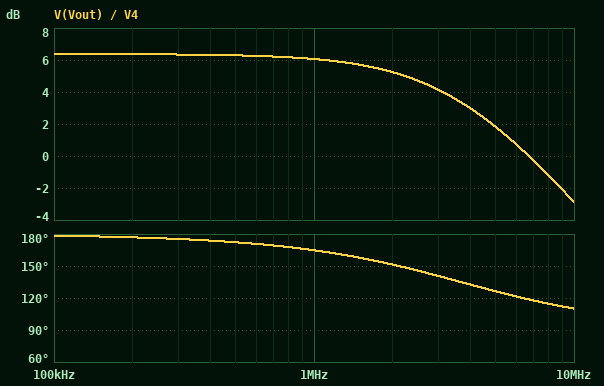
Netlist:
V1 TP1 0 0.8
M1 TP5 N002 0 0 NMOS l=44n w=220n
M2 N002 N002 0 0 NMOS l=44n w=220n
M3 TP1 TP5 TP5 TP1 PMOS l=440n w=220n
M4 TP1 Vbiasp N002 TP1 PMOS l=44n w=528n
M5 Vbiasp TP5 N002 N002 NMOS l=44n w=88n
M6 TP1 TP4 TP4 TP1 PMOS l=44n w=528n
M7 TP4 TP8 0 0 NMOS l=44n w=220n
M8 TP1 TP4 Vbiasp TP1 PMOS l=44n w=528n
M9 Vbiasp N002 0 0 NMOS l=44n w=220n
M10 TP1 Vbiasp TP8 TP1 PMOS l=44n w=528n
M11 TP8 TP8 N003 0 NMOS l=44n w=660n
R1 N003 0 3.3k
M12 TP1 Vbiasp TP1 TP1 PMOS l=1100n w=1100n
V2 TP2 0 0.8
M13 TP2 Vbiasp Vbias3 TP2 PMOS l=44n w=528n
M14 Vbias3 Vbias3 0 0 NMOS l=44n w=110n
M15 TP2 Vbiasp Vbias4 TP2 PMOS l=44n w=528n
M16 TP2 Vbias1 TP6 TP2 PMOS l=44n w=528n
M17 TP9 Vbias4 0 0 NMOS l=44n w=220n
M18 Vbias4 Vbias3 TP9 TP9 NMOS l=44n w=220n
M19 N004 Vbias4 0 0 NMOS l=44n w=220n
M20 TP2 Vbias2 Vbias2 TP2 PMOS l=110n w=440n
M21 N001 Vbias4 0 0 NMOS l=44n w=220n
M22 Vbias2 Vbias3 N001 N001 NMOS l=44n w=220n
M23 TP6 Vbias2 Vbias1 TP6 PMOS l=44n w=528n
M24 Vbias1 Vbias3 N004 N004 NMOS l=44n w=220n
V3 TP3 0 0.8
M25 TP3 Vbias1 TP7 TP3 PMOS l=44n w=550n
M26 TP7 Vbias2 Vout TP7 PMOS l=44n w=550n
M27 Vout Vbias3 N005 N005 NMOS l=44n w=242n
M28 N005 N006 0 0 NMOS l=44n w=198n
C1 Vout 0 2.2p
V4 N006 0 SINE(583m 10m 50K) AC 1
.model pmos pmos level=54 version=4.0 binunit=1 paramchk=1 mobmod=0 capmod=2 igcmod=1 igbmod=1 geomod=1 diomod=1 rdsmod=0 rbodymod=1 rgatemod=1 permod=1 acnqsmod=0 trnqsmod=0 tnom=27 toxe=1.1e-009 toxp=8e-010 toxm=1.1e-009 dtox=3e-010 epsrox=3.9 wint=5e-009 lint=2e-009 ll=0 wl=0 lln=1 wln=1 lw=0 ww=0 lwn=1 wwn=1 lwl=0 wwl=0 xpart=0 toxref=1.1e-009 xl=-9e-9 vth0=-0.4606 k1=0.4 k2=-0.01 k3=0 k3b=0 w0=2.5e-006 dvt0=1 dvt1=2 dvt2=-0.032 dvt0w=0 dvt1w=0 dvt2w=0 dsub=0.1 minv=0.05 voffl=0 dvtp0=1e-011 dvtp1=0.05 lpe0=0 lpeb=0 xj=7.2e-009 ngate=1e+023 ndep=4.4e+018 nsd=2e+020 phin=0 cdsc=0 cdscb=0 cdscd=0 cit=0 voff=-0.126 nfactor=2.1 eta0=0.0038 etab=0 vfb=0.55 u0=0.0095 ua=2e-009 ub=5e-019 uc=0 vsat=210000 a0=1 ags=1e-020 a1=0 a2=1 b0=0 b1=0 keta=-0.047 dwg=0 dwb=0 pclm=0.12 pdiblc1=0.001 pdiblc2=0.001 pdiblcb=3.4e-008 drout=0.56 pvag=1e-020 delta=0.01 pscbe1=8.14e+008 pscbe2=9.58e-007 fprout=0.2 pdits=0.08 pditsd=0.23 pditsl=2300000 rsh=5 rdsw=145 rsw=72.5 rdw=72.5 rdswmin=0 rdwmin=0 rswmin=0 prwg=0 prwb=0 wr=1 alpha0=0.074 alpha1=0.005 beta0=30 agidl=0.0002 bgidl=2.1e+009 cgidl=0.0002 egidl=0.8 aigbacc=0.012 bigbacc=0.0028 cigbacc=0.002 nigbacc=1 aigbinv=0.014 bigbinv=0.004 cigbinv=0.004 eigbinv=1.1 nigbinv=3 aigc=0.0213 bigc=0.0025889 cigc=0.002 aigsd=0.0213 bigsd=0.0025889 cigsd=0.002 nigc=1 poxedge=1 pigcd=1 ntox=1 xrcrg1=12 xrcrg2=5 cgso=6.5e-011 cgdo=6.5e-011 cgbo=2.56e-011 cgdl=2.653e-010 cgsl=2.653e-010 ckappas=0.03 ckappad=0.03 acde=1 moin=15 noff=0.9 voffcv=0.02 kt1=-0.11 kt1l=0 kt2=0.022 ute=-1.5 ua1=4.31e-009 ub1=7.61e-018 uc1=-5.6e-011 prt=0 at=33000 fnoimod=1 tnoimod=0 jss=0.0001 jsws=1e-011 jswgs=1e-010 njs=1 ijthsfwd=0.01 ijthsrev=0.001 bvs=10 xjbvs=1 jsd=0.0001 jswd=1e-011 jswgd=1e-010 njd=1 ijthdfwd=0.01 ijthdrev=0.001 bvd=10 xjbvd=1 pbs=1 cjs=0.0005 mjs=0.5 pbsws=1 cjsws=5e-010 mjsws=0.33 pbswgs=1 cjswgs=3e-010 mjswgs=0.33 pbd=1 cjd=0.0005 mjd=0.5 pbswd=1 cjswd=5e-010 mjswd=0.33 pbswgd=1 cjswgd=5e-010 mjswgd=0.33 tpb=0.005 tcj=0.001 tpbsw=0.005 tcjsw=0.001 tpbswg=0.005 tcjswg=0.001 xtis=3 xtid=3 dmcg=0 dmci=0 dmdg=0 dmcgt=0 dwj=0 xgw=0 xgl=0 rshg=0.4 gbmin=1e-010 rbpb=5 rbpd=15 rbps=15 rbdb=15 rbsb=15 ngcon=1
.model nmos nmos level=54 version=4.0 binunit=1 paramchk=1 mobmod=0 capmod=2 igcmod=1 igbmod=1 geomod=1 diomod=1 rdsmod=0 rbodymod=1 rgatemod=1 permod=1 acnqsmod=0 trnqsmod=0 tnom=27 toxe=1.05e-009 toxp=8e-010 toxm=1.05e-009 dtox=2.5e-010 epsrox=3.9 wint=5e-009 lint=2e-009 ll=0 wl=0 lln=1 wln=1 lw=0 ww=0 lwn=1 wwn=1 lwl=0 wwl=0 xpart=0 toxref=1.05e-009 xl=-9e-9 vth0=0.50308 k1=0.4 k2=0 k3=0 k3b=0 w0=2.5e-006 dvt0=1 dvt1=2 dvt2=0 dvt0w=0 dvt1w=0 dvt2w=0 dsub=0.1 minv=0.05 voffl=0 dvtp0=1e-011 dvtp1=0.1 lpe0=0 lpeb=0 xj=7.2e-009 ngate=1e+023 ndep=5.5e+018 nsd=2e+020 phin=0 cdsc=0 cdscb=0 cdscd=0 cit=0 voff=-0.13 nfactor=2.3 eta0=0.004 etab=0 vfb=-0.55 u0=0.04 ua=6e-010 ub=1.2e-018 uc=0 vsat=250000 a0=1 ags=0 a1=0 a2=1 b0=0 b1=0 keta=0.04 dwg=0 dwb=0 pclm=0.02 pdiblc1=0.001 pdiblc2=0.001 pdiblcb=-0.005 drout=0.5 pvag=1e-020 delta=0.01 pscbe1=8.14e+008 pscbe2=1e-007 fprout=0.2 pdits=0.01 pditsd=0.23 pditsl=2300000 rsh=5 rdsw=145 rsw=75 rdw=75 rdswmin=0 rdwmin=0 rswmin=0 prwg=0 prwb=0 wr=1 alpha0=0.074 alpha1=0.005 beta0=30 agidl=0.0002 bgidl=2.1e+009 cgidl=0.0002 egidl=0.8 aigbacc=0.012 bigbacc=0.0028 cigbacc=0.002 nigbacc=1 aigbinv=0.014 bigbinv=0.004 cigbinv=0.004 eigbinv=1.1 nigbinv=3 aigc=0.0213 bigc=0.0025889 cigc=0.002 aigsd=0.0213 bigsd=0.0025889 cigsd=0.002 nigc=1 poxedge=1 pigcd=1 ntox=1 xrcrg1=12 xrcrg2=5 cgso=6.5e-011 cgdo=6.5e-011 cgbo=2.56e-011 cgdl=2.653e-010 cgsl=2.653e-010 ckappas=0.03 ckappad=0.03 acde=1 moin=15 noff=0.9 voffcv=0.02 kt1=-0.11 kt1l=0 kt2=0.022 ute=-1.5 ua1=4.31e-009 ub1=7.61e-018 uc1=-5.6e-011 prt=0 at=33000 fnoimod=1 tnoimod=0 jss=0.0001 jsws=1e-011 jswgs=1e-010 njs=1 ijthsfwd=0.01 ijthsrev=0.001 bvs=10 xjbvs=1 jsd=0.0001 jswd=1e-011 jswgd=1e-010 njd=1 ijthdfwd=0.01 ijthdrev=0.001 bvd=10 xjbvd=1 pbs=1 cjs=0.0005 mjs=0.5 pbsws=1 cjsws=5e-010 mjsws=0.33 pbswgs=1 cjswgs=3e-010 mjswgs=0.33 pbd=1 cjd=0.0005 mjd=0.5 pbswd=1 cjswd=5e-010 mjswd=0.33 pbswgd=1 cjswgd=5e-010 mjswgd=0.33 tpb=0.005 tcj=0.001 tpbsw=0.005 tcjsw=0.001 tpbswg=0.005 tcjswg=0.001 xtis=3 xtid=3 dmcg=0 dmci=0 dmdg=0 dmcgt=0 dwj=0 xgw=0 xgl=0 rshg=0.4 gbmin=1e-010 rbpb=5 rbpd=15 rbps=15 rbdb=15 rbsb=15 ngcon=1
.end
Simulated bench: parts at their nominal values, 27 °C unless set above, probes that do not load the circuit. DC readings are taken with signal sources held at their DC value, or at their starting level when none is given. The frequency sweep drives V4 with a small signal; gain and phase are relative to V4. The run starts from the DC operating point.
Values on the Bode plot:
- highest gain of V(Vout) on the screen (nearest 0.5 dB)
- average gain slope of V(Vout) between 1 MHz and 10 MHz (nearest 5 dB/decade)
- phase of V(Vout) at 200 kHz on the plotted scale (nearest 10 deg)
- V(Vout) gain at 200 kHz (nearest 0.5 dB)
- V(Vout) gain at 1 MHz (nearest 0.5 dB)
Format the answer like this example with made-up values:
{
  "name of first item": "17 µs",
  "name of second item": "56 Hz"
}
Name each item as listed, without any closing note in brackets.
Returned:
{
  "highest gain of V(Vout) on the screen": "6.5 dB",
  "average gain slope of V(Vout) between 1 MHz and 10 MHz": "-10 dB/decade",
  "phase of V(Vout) at 200 kHz on the plotted scale": "180 deg",
  "V(Vout) gain at 200 kHz": "6.5 dB",
  "V(Vout) gain at 1 MHz": "6.0 dB"
}
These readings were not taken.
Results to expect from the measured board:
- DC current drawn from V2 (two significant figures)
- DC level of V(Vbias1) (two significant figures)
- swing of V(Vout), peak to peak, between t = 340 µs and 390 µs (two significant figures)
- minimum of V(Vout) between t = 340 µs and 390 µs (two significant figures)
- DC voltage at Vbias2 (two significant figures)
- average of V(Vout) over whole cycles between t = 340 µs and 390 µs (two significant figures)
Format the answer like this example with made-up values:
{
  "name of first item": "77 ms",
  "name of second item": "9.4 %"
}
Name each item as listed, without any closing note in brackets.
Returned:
{
  "DC current drawn from V2": "61 µA",
  "DC level of V(Vbias1)": "190 mV",
  "swing of V(Vout), peak to peak, between t = 340 µs and 390 µs": "42 mV",
  "minimum of V(Vout) between t = 340 µs and 390 µs": "640 mV",
  "DC voltage at Vbias2": "95 mV",
  "average of V(Vout) over whole cycles between t = 340 µs and 390 µs": "660 mV"
}
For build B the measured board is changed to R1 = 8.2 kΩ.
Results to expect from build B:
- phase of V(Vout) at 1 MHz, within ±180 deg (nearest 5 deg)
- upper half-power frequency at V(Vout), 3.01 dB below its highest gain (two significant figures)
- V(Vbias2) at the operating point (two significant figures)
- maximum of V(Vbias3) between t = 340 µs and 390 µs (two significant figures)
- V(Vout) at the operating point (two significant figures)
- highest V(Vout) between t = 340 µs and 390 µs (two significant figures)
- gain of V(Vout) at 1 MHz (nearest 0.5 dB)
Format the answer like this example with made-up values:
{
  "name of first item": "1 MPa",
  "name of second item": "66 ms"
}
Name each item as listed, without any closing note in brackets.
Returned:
{
  "phase of V(Vout) at 1 MHz, within ±180 deg": "140 deg",
  "upper half-power frequency at V(Vout), 3.01 dB below its highest gain": "1.2 MHz",
  "V(Vbias2) at the operating point": "180 mV",
  "maximum of V(Vbias3) between t = 340 µs and 390 µs": "560 mV",
  "V(Vout) at the operating point": "110 mV",
  "highest V(Vout) between t = 340 µs and 390 µs": "130 mV",
  "gain of V(Vout) at 1 MHz": "0.5 dB"
}
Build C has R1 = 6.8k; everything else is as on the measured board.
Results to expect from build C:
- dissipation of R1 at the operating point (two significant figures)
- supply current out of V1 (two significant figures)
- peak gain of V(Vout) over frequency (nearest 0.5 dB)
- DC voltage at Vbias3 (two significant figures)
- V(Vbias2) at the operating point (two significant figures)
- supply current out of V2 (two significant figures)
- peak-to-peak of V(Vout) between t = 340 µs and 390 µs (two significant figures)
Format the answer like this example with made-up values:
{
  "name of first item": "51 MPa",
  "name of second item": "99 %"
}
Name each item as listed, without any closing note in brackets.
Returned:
{
  "dissipation of R1 at the operating point": "370 nW",
  "supply current out of V1": "30 µA",
  "peak gain of V(Vout) over frequency": "15.5 dB",
  "DC voltage at Vbias3": "570 mV",
  "V(Vbias2) at the operating point": "160 mV",
  "supply current out of V2": "28 µA",
  "peak-to-peak of V(Vout) between t = 340 µs and 390 µs": "150 mV"
}
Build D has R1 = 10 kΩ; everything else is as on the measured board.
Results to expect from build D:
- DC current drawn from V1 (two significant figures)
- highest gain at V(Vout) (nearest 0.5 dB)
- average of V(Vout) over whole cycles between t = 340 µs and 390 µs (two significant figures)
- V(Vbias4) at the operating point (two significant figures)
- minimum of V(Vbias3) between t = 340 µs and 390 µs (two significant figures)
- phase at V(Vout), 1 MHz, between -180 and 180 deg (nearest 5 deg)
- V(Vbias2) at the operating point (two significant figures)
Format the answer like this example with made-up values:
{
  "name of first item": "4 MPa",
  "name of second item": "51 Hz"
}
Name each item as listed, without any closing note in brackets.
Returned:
{
  "DC current drawn from V1": "20 µA",
  "highest gain at V(Vout)": "-3.0 dB",
  "average of V(Vout) over whole cycles between t = 340 µs and 390 µs": "86 mV",
  "V(Vbias4) at the operating point": "530 mV",
  "minimum of V(Vbias3) between t = 340 µs and 390 µs": "540 mV",
  "phase at V(Vout), 1 MHz, between -180 and 180 deg": "150 deg",
  "V(Vbias2) at the operating point": "200 mV"
}
